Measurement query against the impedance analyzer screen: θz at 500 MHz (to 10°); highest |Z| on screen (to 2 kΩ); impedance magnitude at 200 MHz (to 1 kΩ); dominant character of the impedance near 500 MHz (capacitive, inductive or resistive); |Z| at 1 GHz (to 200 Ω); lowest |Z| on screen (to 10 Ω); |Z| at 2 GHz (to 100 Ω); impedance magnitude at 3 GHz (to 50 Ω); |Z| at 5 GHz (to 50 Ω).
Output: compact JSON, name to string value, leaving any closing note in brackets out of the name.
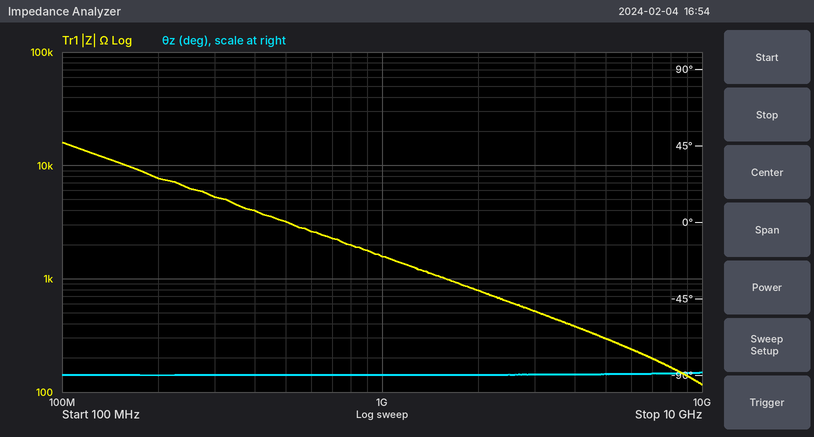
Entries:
{"θz at 500 MHz": "-90°", "highest |Z| on screen": "16 kΩ", "impedance magnitude at 200 MHz": "8 kΩ", "dominant character of the impedance near 500 MHz": "capacitive", "|Z| at 1 GHz": "1.6 kΩ", "lowest |Z| on screen": "120 Ω", "|Z| at 2 GHz": "800 Ω", "impedance magnitude at 3 GHz": "500 Ω", "|Z| at 5 GHz": "300 Ω"}
